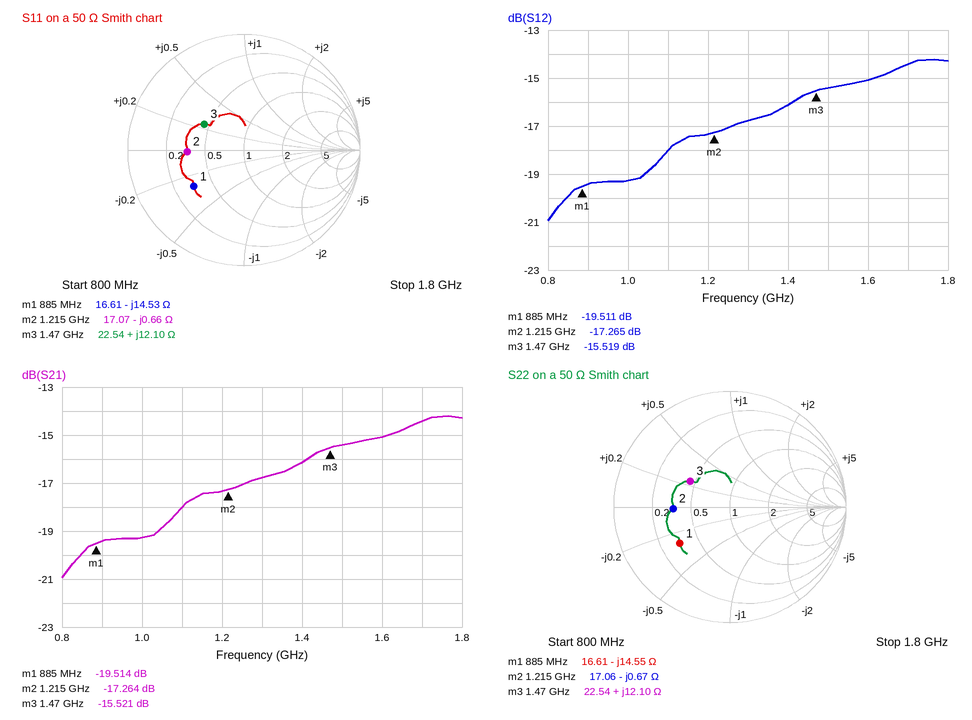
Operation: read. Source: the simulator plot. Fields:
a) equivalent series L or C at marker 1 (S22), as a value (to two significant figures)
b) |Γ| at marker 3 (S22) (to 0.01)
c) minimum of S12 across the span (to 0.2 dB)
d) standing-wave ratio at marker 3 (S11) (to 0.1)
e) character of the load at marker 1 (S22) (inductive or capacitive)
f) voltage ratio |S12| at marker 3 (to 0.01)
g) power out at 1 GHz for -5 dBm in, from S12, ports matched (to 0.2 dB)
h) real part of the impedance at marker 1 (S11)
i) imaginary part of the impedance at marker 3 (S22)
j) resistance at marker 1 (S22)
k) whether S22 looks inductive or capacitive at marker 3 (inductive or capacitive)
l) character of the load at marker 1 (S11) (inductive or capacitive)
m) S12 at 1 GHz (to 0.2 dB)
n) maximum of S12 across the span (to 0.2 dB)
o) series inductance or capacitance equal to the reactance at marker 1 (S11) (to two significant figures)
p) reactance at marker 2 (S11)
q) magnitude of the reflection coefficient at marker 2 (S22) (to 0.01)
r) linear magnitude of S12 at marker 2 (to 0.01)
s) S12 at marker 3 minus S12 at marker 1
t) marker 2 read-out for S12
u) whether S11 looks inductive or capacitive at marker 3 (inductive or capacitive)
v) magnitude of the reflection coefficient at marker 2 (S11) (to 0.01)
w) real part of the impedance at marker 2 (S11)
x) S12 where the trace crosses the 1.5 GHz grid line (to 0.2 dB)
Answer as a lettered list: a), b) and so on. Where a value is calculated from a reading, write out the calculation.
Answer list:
a) C = 1/(2π × 885 MHz × 14.55 Ω) ≈ 12 pF
b) 0.41
c) -21.0 dB
d) 2.4
e) capacitive
f) 10^(-15.519/20) ≈ 0.17
g) -5 dBm + (-19.2 dB) = -24.2 dBm
h) 16.61 Ω
i) +12.10 Ω
j) 16.61 Ω
k) inductive
l) capacitive
m) -19.2 dB
n) -14.2 dB
o) C = 1/(2π × 885 MHz × 14.53 Ω) ≈ 12 pF
p) -0.66 Ω
q) 0.49
r) 10^(-17.265/20) ≈ 0.14
s) -15.519 − (-19.511) = 3.992 dB
t) -17.265 dB
u) inductive
v) 0.49
w) 17.07 Ω
x) -15.4 dB
